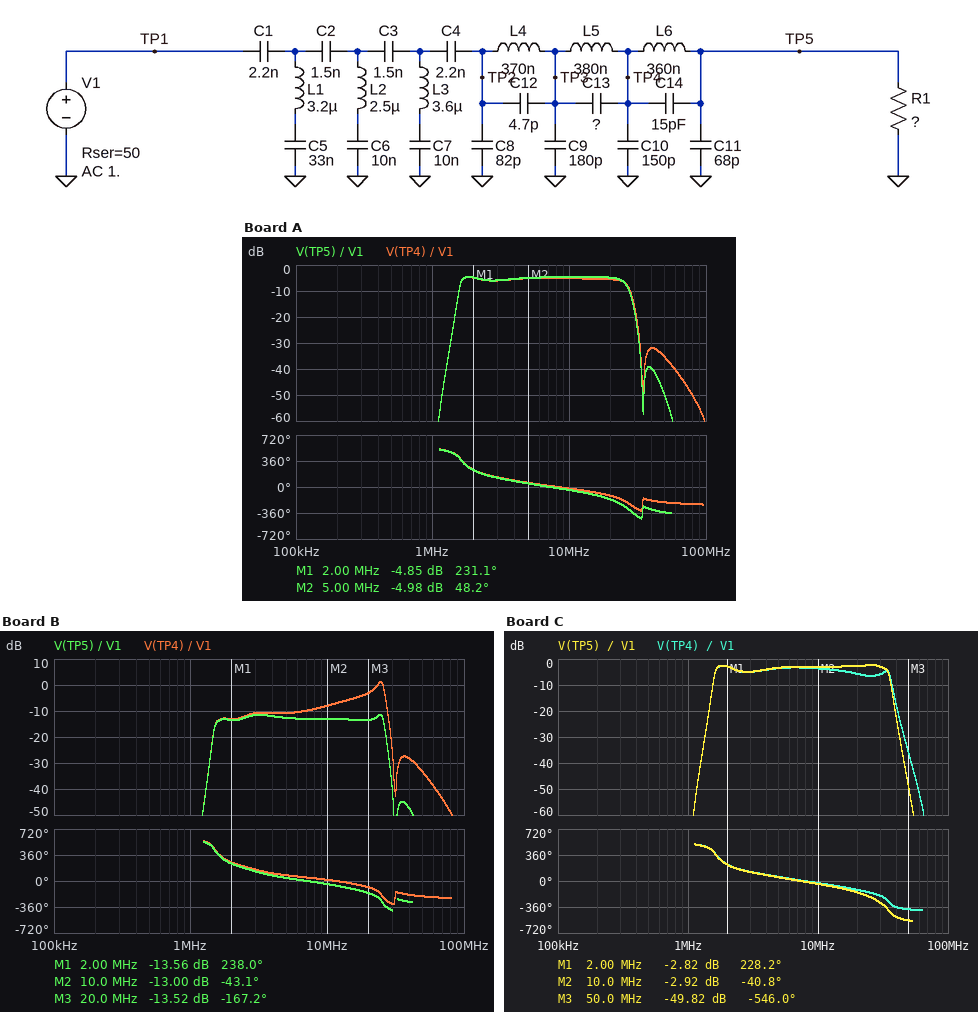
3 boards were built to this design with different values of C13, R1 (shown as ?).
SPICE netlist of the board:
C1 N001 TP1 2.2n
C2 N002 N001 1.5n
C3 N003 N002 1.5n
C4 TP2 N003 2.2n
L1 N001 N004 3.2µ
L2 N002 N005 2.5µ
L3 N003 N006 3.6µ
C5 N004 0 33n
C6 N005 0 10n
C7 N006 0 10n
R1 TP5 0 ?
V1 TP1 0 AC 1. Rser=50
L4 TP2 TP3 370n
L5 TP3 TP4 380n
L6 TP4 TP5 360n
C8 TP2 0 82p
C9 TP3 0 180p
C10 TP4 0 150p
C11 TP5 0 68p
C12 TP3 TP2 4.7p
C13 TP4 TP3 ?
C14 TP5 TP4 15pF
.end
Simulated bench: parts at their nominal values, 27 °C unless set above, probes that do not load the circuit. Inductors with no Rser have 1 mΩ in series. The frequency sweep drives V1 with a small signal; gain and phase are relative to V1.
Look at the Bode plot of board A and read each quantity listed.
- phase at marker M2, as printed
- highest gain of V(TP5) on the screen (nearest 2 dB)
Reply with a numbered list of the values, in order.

1. 48.2 deg
2. -4 dB
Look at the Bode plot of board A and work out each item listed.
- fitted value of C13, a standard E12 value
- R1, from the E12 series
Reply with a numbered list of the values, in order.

1. 56 pF
2. 68 Ω
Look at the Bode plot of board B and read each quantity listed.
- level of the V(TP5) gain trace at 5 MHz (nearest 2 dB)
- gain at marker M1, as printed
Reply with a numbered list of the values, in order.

1. -12 dB
2. -13.56 dB
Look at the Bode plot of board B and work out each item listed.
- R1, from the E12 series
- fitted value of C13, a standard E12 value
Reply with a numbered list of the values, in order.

1. 15 Ω
2. 68 pF
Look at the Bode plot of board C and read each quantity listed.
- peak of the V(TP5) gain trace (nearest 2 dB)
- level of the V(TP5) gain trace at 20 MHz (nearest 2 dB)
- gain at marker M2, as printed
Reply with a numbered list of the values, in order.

1. -2 dB
2. -2 dB
3. -2.92 dB
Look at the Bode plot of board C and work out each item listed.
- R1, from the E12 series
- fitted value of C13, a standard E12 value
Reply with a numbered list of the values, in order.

1. 120 Ω
2. 12 pF
